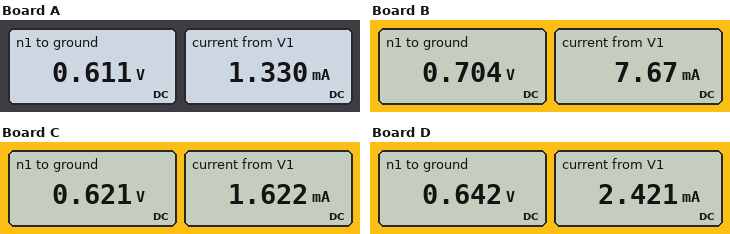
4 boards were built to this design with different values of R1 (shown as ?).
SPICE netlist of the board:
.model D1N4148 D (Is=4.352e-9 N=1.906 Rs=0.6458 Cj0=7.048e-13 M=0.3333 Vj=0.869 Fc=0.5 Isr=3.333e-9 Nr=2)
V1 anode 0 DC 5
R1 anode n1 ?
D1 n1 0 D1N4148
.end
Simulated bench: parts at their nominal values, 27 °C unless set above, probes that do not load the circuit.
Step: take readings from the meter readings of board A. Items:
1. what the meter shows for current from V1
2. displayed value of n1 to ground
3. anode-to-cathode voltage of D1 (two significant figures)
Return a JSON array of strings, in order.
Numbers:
["1.330 mA", "0.611 V", "610 mV"]
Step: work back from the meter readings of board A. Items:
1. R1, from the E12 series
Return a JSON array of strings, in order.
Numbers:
["3.3 kΩ"]
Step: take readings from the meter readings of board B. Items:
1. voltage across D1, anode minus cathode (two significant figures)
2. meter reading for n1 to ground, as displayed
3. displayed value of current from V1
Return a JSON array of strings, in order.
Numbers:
["700 mV", "0.704 V", "7.67 mA"]
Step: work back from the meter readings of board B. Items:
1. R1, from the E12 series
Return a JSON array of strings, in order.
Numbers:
["560 Ω"]
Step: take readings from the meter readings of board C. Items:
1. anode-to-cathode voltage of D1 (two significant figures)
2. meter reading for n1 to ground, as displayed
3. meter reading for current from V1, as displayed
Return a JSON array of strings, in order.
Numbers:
["620 mV", "0.621 V", "1.622 mA"]
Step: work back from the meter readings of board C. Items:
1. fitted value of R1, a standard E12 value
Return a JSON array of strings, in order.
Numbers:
["2.7 kΩ"]
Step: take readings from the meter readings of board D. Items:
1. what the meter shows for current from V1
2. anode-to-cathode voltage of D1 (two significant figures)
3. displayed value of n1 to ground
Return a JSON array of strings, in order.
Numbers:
["2.421 mA", "640 mV", "0.642 V"]
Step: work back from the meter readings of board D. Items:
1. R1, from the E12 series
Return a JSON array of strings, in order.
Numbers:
["1.8 kΩ"]
